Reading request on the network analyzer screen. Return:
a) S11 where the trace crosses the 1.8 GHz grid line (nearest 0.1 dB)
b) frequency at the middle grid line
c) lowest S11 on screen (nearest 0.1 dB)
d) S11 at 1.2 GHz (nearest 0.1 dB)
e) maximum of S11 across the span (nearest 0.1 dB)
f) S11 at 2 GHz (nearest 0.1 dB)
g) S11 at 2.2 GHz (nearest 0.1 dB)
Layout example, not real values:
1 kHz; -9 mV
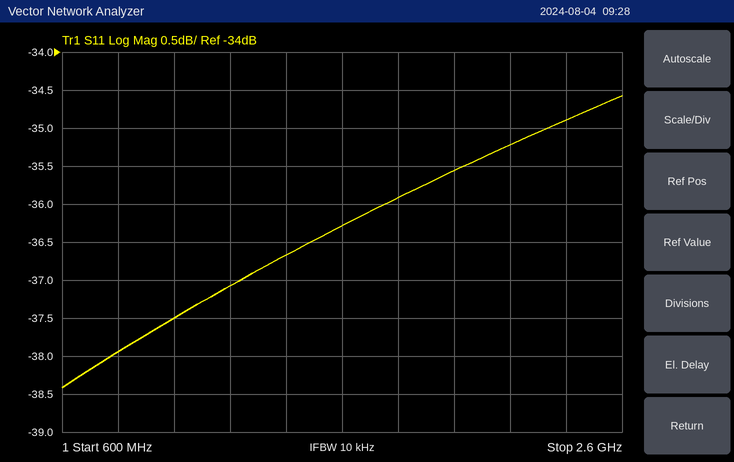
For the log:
-35.9 dB; 1.6 GHz; -38.4 dB; -37.1 dB; -34.6 dB; -35.6 dB; -35.2 dB
